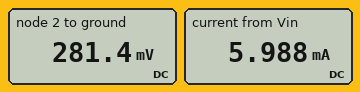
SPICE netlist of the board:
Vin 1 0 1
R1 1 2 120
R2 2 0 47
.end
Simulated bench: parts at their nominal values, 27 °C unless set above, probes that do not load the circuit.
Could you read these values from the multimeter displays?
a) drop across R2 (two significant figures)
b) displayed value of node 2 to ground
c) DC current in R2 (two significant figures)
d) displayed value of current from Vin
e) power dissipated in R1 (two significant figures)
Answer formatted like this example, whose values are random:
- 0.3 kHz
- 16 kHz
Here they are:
- 280 mV
- 281.4 mV
- 6.0 mA
- 5.988 mA
- 4.3 mW
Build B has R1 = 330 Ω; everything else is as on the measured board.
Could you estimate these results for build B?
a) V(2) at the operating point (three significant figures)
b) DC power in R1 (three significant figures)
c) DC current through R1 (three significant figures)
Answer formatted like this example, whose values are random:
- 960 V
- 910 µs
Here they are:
- 125 mV
- 2.32 mW
- 2.65 mA
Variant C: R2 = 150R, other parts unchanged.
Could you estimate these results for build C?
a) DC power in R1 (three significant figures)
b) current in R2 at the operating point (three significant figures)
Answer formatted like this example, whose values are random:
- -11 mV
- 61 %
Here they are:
- 1.65 mW
- 3.70 mA
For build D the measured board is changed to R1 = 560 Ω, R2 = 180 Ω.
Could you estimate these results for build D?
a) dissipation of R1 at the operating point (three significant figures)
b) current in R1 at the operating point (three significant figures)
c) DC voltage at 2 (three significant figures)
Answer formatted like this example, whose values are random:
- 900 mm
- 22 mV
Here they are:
- 1.02 mW
- 1.35 mA
- 243 mV
